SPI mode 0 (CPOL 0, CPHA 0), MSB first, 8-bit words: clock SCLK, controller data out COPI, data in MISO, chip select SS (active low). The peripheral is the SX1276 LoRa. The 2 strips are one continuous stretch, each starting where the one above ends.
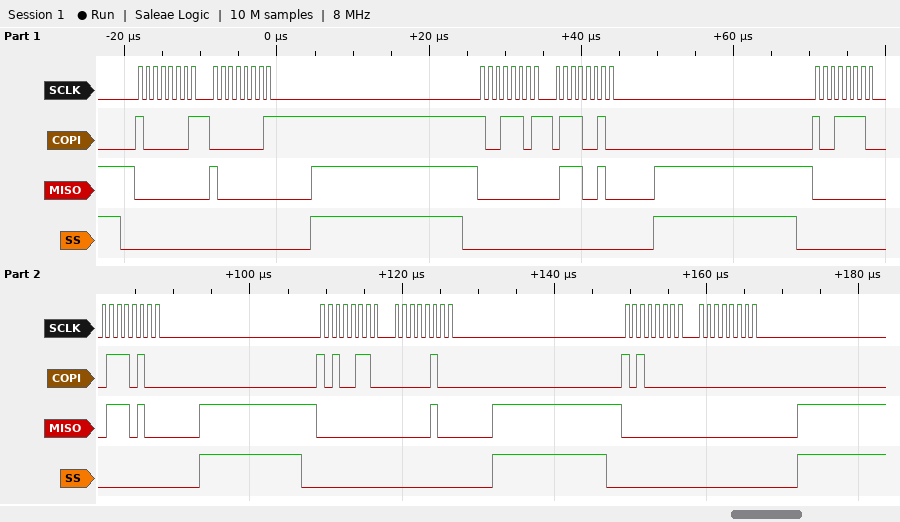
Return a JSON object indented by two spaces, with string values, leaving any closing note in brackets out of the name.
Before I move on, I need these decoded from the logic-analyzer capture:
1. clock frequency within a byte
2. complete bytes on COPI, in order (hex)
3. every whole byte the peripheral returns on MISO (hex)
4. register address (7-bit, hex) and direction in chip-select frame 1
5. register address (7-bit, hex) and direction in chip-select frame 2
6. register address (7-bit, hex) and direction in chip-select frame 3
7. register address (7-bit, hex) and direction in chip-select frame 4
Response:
{
  "clock frequency within a byte": "1 MHz",
  "complete bytes on COPI, in order": "81 01 9D 72 9E 74 A6 04 A0 00",
  "every whole byte the peripheral returns on MISO": "00 80 00 72 00 74 00 04 00 00",
  "register address (7-bit, hex) and direction in chip-select frame 1": "0x01 write",
  "register address (7-bit, hex) and direction in chip-select frame 2": "0x1D write",
  "register address (7-bit, hex) and direction in chip-select frame 3": "0x1E write",
  "register address (7-bit, hex) and direction in chip-select frame 4": "0x26 write"
}
